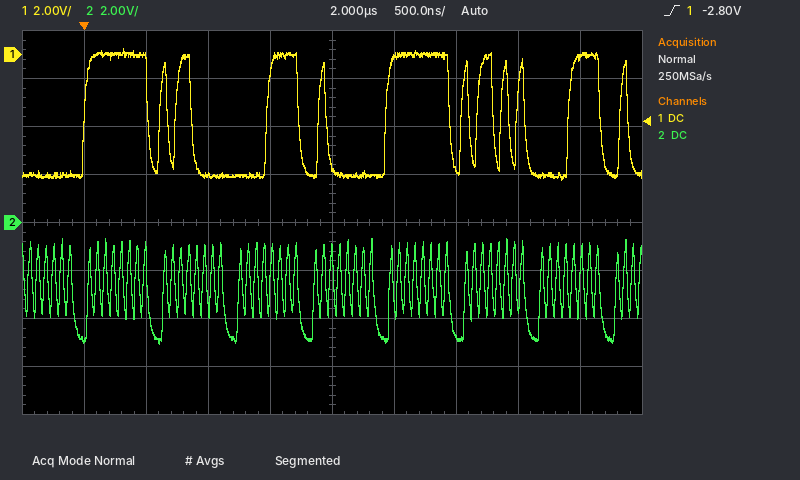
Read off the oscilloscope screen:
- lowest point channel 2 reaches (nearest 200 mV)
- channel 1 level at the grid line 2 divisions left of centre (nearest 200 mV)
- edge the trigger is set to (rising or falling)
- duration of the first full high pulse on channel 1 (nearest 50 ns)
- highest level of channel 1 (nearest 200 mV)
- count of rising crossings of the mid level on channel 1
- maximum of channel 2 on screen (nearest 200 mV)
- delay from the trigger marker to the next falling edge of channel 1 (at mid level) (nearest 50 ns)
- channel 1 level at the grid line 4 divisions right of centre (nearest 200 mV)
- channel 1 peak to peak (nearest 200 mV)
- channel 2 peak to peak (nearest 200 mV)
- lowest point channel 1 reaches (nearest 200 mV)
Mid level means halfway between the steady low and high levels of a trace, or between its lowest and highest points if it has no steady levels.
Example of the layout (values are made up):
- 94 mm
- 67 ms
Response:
- -5.0 V
- -5.0 V
- rising
- 500 ns
- 200 mV
- 12
- -600 mV
- 500 ns
- 0.0 V
- 5.4 V
- 4.4 V
- -5.2 V
